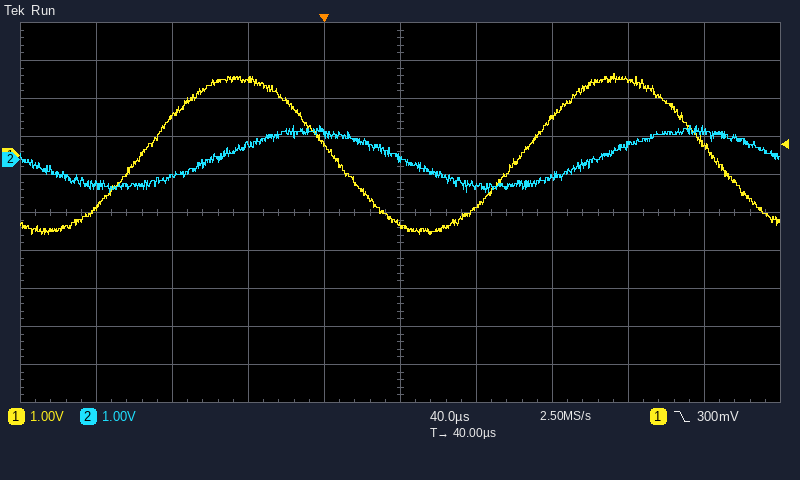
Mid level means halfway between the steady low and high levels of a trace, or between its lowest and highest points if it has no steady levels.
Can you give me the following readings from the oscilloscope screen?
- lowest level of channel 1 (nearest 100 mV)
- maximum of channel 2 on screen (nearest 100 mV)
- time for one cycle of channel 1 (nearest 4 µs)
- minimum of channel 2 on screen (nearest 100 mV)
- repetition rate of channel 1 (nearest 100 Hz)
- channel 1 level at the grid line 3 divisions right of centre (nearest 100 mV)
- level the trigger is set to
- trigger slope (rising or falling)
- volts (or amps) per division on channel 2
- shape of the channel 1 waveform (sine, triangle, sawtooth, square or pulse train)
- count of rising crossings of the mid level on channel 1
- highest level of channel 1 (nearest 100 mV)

-2.1 V
900 mV
200 µs
-900 mV
5.0 kHz
2.0 V
300 mV
falling
1 V
sine
2
2.2 V
